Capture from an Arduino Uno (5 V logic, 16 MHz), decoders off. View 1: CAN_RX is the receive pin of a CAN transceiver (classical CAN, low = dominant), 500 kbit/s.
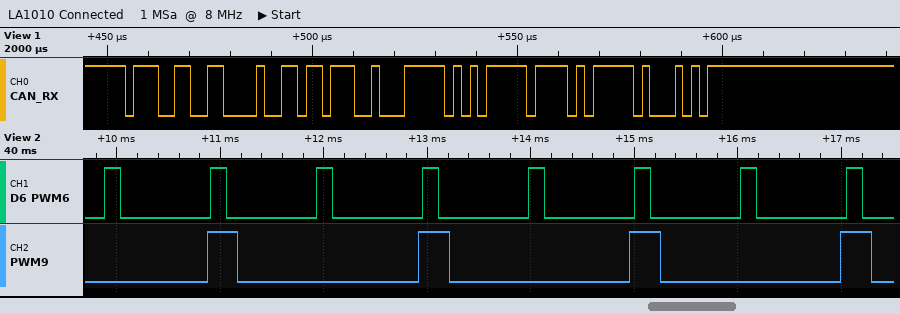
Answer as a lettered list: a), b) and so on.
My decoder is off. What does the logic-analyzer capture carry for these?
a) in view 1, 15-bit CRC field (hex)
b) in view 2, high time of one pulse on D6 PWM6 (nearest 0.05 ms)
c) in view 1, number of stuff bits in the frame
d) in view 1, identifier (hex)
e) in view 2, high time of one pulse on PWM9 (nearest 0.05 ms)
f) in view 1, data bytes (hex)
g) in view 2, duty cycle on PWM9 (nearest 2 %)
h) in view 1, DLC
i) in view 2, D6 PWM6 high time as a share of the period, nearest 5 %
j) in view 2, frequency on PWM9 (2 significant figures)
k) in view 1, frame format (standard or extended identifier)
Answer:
a) 0x57E2
b) 0.15 ms
c) 3
d) 0x733
e) 0.30 ms
f) DB 91 FA FF
g) 14 %
h) 4
i) 15 %
j) 490 Hz
k) standard
